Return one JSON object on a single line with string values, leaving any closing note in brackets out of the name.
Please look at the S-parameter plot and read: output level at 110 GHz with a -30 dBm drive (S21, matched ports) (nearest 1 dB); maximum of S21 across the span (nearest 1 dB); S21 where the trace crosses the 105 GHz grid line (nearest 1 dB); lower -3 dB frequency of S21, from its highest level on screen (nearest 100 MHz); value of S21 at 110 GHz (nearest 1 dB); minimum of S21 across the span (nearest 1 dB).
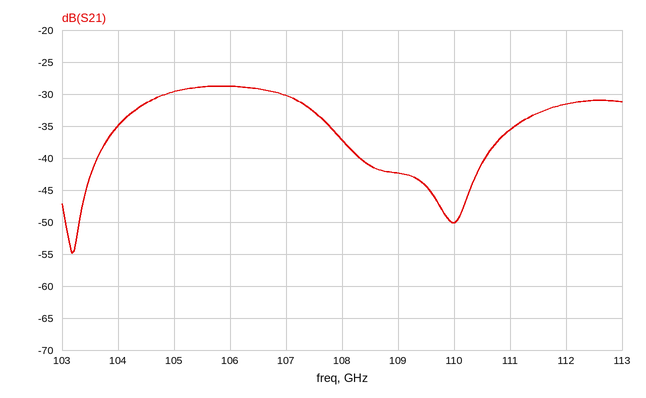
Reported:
{"output level at 110 GHz with a -30 dBm drive (S21, matched ports)": "-80 dBm", "maximum of S21 across the span": "-29 dB", "S21 where the trace crosses the 105 GHz grid line": "-30 dB", "lower -3 dB frequency of S21, from its highest level on screen": "104.4 GHz", "value of S21 at 110 GHz": "-50 dB", "minimum of S21 across the span": "-55 dB"}
